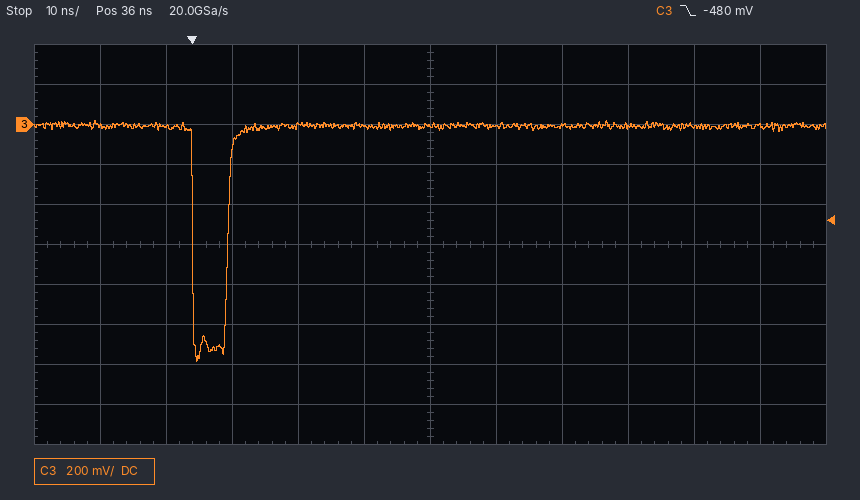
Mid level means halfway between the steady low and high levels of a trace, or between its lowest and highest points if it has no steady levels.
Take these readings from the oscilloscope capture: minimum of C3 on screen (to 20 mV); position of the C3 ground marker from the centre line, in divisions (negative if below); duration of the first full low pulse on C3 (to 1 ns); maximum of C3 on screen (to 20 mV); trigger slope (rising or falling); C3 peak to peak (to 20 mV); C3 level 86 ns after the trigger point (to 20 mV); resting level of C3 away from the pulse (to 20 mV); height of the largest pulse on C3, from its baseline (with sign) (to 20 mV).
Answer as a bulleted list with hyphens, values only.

- -1.18 V
- +3.0 div
- 5 ns
- 20 mV
- falling
- 1.20 V
- 0 mV
- 0 mV
- -1.18 V
